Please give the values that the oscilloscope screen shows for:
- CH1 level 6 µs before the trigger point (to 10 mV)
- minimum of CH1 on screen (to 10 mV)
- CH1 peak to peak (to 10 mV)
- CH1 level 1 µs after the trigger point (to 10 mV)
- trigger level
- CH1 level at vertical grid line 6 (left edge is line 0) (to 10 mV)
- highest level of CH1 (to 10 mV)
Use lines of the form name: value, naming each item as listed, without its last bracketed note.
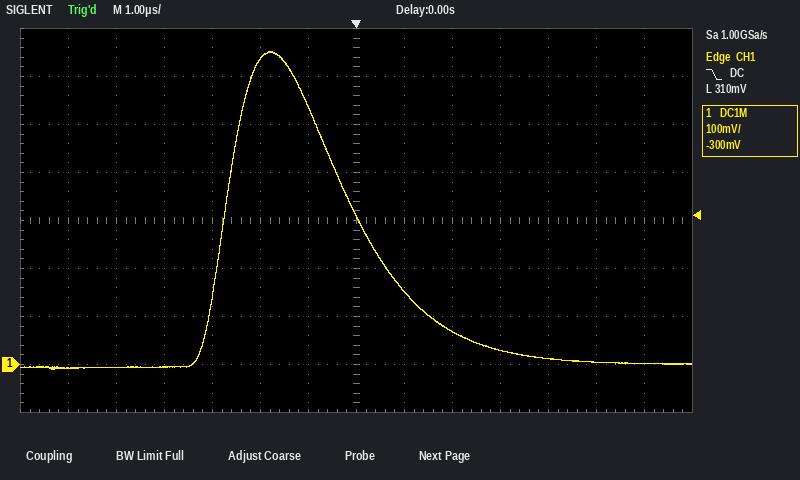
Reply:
CH1 level 6 µs before the trigger point: -10 mV
minimum of CH1 on screen: -10 mV
CH1 peak to peak: 660 mV
CH1 level 1 µs after the trigger point: 150 mV
trigger level: 310 mV
CH1 level at vertical grid line 6 (left edge is line 0): 540 mV
highest level of CH1: 650 mV
